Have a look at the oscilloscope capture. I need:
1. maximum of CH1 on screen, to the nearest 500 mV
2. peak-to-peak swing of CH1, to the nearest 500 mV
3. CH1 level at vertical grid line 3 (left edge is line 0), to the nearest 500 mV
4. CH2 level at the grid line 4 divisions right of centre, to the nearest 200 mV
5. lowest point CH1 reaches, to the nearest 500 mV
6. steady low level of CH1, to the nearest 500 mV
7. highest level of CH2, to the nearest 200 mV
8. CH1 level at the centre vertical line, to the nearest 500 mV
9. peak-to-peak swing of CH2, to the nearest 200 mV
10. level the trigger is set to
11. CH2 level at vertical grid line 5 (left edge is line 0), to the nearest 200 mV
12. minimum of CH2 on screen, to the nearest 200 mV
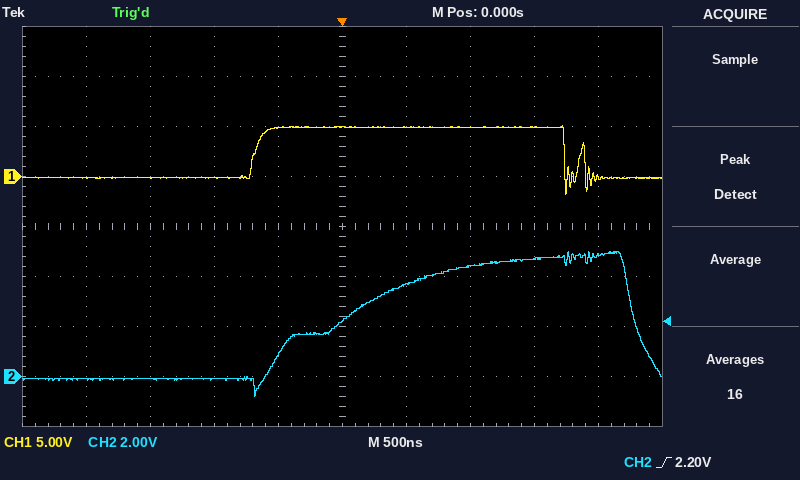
5.0 V
7.0 V
0.0 V
4.8 V
-2.0 V
0.0 V
5.0 V
5.0 V
5.8 V
2.20 V
2.2 V
-800 mV
